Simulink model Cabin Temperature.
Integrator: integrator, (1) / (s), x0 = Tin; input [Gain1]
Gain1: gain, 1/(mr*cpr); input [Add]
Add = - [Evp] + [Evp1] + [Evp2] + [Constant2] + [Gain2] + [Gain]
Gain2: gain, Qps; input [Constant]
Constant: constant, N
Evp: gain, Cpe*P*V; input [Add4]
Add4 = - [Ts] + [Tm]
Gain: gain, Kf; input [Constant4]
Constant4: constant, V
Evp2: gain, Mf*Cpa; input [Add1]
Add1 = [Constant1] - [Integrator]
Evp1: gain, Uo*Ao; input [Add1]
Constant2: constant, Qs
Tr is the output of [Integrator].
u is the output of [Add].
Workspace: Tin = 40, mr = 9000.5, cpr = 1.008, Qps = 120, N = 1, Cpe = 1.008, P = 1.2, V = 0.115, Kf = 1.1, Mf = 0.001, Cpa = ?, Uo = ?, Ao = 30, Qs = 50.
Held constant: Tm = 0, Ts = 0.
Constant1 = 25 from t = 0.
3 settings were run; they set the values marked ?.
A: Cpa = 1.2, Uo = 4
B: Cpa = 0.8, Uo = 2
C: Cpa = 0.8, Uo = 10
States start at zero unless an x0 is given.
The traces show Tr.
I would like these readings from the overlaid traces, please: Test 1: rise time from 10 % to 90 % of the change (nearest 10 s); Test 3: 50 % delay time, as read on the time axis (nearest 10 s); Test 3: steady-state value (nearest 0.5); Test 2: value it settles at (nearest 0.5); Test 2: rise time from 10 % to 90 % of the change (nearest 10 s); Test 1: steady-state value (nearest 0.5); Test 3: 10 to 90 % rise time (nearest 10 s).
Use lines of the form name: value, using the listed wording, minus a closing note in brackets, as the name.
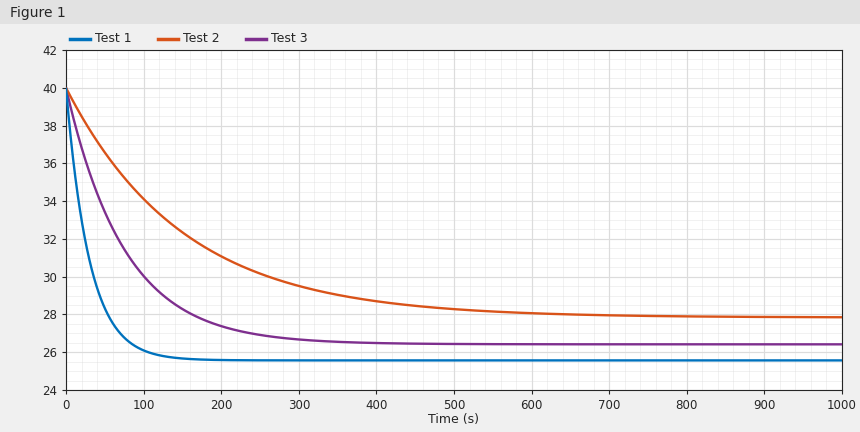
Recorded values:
Test 1: rise time from 10 % to 90 % of the change: 70 s
Test 3: 50 % delay time, as read on the time axis: 50 s
Test 3: steady-state value: 26.5
Test 2: value it settles at: 28.0
Test 2: rise time from 10 % to 90 % of the change: 330 s
Test 1: steady-state value: 25.5
Test 3: 10 to 90 % rise time: 170 s
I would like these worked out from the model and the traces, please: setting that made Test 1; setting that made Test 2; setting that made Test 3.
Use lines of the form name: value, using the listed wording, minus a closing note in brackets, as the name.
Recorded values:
setting that made Test 1: C
setting that made Test 2: B
setting that made Test 3: A
